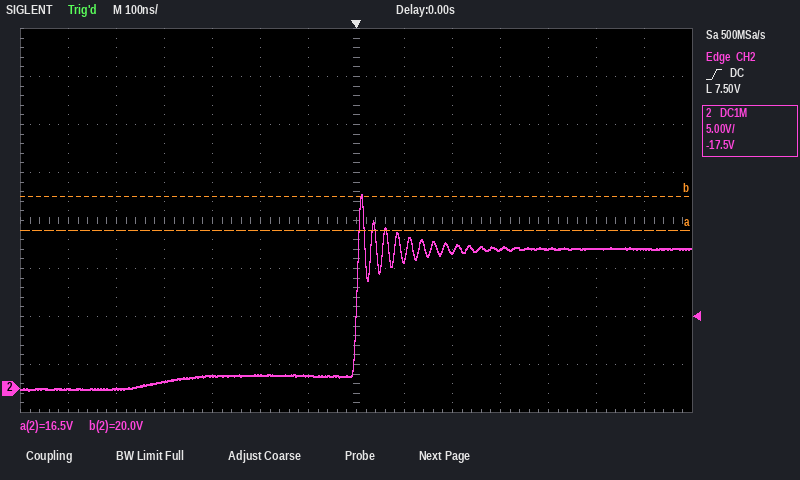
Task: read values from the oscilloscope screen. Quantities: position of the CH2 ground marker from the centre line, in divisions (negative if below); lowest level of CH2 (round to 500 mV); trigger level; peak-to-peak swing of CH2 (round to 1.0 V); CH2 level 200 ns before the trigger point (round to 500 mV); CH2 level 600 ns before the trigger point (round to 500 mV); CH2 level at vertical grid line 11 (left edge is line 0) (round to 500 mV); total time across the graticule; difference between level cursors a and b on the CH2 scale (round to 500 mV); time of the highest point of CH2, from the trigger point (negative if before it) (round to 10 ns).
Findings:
-3.5 div
0.0 V
7.50 V
20.0 V
1.5 V
0.0 V
14.5 V
1.4 µs
3.5 V
+10 ns
